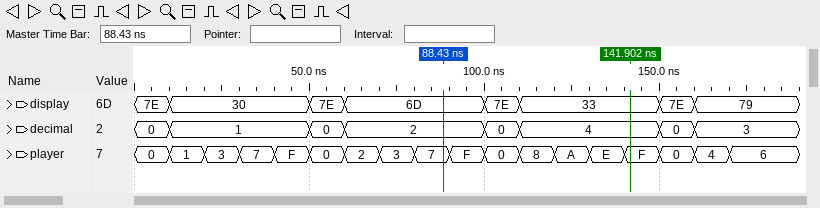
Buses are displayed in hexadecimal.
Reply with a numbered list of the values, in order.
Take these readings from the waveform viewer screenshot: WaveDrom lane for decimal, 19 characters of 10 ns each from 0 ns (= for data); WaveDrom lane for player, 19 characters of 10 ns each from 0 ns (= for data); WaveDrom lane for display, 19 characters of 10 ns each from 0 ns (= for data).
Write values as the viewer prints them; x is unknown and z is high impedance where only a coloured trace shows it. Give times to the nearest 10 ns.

1. {name: 'decimal', wave: '==...==...==...==..', data: '0 1 0 2 0 4 0 3'}
2. {name: 'player', wave: '==================.', data: '0 1 3 7 F 0 2 3 7 F 0 8 A E F 0 4 6'}
3. {name: 'display', wave: '==...==...==...==..', data: '7E 30 7E 6D 7E 33 7E 79'}
